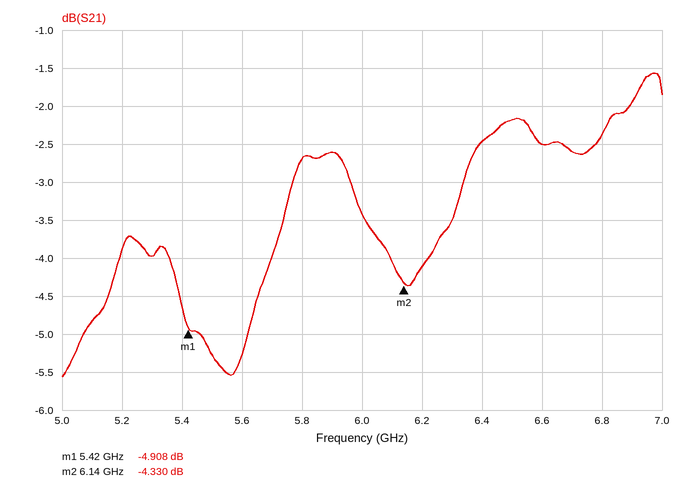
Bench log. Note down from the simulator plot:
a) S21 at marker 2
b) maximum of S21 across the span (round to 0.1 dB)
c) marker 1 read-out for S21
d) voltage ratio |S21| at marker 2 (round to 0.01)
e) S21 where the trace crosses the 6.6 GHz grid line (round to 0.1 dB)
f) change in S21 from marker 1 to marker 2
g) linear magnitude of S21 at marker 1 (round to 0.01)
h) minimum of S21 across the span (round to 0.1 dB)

-4.330 dB
-1.6 dB
-4.908 dB
0.61
-2.5 dB
0.578 dB
0.57
-5.6 dB
